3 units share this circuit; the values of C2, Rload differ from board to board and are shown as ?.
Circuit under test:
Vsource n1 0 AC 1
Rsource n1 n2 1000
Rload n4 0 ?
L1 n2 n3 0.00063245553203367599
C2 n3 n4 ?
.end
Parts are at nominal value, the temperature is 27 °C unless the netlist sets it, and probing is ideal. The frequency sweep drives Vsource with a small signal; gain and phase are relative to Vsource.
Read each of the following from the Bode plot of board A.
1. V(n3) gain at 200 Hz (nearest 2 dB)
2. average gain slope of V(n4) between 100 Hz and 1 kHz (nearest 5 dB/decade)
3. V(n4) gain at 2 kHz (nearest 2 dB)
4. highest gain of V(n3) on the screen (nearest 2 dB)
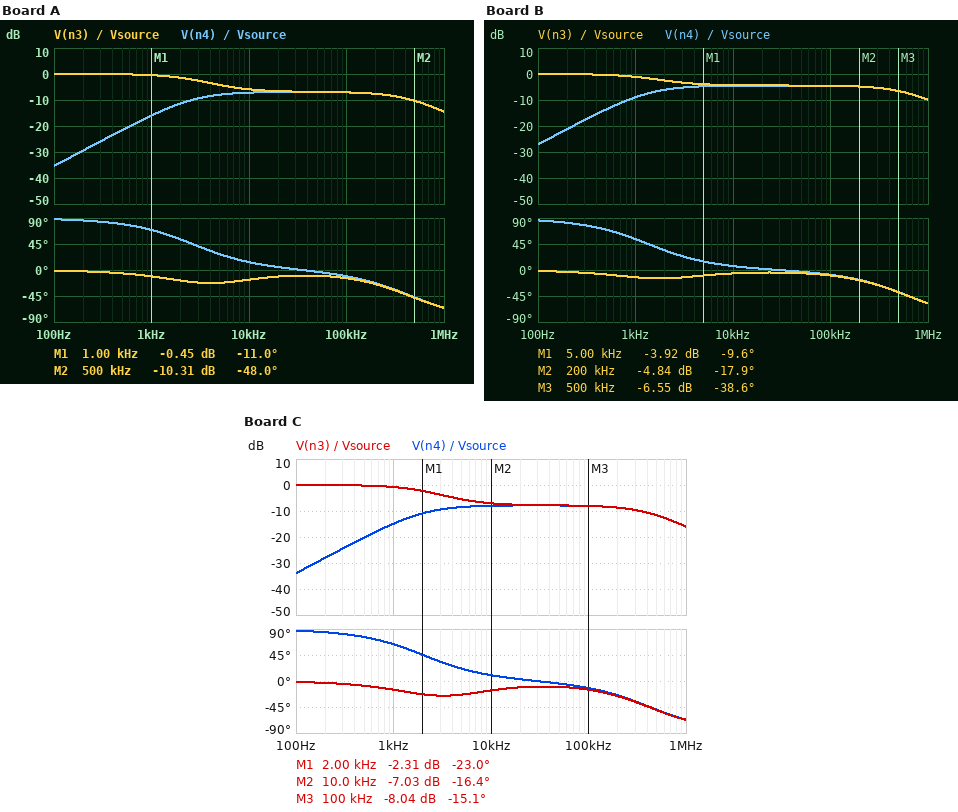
0 dB
20 dB/decade
-12 dB
0 dB
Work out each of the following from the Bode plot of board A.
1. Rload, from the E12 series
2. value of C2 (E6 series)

820 Ω
33 nF
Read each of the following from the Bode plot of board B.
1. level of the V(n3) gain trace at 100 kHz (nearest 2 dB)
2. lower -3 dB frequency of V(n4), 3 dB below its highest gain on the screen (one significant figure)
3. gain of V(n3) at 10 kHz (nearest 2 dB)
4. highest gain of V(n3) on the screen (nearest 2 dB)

-4 dB
1 kHz
-4 dB
0 dB
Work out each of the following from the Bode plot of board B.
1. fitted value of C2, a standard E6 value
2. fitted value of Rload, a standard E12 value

47 nF
1.5 kΩ
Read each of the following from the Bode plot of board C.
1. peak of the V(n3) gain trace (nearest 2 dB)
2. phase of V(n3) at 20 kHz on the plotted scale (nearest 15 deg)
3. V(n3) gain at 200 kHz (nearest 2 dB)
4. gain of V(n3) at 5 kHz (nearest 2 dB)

0 dB
-15 deg
-8 dB
-6 dB
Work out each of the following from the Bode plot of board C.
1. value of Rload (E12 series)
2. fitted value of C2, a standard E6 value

680 Ω
47 nF
